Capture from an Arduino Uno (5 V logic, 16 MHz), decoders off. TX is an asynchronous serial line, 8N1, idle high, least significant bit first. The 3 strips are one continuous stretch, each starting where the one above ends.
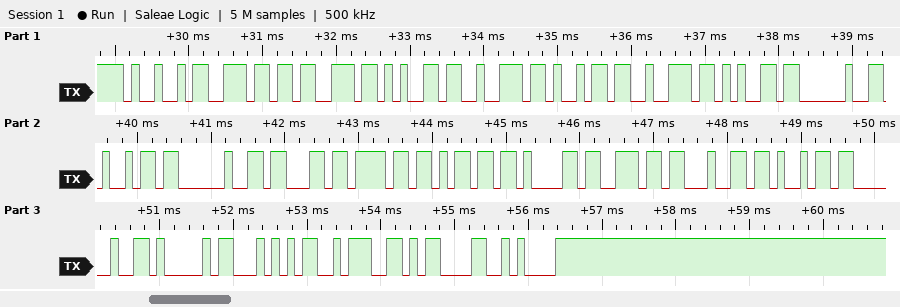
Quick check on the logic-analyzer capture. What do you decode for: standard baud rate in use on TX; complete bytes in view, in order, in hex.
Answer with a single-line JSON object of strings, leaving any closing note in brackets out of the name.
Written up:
{"standard baud rate in use on TX": "9600 baud", "complete bytes in view, in order, in hex": "0x49 0x6E 0x73 0x65 0x72 0x69 0x72 0x65 0x20 0x69 0x20 0x63 0x6F 0x6D 0x61 0x6E 0x64 0x69 0x20 0x41 0x54 0x3A 0x0D 0x0A"}
